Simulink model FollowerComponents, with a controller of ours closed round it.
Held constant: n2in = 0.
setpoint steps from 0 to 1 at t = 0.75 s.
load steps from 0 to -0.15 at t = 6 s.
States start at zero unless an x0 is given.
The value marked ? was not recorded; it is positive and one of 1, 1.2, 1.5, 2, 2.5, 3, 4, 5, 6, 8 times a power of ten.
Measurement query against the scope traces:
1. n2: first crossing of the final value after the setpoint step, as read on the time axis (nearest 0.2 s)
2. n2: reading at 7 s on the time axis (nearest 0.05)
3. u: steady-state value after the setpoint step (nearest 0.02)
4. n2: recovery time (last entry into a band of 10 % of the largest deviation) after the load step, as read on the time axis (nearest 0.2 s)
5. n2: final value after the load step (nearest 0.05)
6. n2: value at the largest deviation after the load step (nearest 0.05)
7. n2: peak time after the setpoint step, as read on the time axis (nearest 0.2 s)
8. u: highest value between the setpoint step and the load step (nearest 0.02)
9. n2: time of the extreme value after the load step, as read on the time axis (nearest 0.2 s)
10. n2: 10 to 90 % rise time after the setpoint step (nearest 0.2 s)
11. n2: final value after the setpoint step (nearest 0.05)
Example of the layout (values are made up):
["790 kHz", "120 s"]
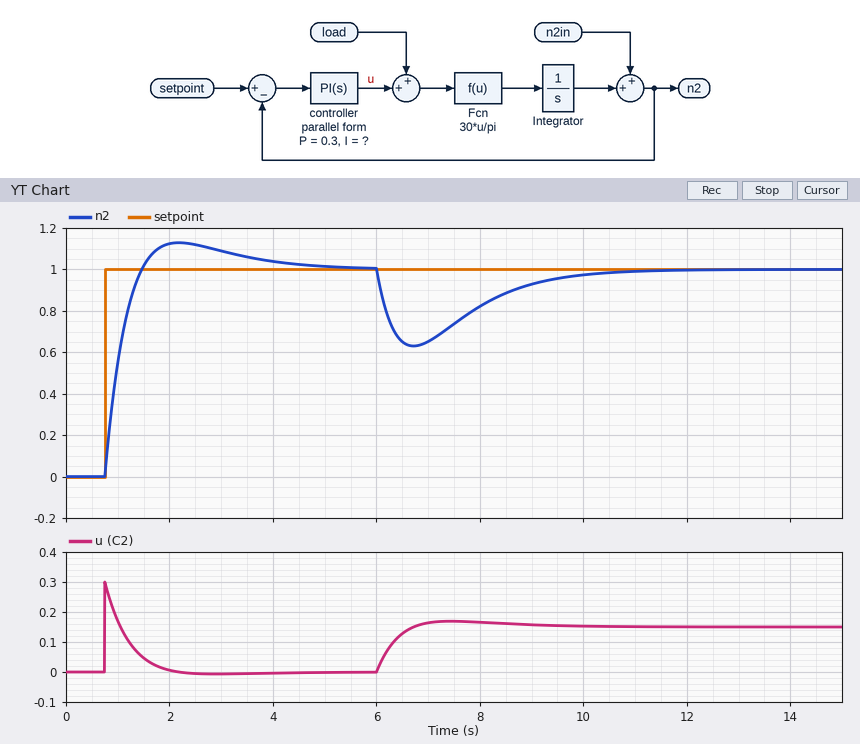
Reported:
["1.4 s", "0.65", "0.00", "9.6 s", "1.00", "0.65", "2.2 s", "0.30", "6.8 s", "0.6 s", "1.00"]
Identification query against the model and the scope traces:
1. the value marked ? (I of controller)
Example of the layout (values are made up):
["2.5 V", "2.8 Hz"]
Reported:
["0.2"]
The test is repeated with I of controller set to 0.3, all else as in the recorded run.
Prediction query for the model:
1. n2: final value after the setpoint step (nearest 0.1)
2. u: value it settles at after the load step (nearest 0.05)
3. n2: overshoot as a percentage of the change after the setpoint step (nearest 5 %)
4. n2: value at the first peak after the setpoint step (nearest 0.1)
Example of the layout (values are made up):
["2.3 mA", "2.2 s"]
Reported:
["1.0", "0.15", "15 %", "1.2"]
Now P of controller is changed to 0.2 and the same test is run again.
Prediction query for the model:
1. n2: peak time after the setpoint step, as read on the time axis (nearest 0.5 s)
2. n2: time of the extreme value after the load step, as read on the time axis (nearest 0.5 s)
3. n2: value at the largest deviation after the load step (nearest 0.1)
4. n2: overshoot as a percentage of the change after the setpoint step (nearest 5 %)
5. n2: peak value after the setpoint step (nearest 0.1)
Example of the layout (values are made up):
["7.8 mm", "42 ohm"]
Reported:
["2.5 s", "7.0 s", "0.5", "20 %", "1.2"]
